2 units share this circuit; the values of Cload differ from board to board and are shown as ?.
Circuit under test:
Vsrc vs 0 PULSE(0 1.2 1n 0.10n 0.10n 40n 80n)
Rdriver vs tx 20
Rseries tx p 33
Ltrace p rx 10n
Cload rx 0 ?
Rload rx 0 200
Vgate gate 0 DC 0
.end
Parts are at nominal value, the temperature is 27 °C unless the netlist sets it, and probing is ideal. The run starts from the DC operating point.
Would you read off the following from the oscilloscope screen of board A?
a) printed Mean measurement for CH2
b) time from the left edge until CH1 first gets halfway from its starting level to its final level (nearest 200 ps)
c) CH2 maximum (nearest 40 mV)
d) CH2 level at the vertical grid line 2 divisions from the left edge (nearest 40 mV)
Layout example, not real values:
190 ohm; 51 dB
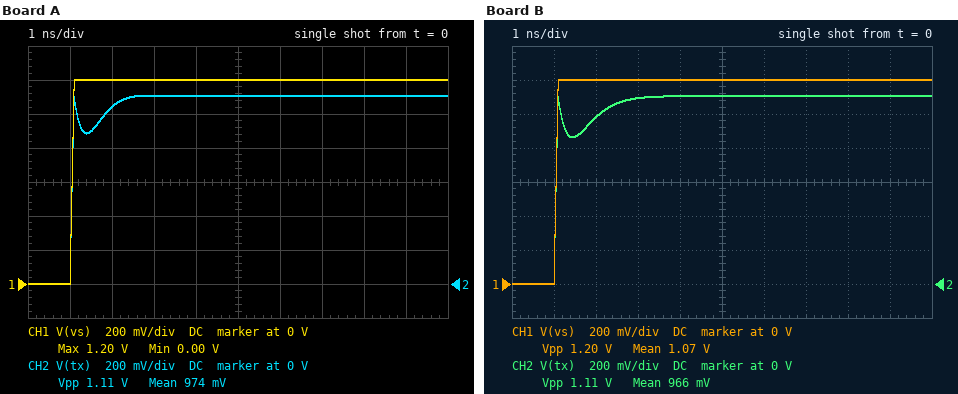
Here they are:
974 mV; 1.0 ns; 1.12 V; 1.04 V
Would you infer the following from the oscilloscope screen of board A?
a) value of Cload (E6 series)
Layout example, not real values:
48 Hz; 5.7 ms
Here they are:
10 pF
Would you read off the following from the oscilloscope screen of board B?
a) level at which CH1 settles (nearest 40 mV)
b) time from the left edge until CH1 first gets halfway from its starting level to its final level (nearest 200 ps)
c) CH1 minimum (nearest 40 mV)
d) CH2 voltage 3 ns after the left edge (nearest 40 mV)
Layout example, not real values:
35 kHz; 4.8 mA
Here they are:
1.20 V; 1.0 ns; 0 V; 1.08 V
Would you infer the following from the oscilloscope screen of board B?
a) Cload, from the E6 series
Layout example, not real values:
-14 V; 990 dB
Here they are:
15 pF
